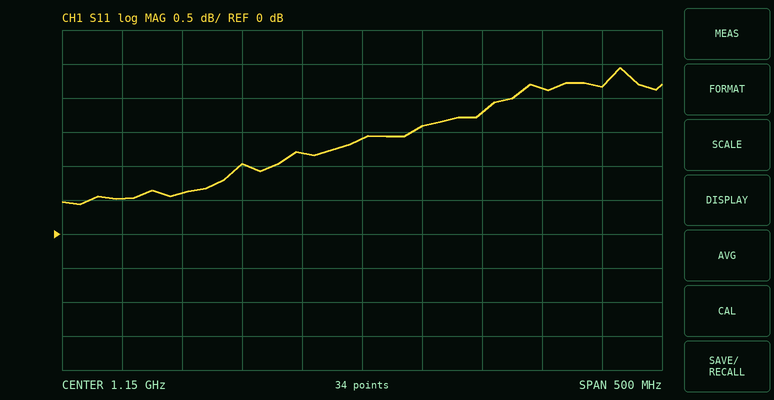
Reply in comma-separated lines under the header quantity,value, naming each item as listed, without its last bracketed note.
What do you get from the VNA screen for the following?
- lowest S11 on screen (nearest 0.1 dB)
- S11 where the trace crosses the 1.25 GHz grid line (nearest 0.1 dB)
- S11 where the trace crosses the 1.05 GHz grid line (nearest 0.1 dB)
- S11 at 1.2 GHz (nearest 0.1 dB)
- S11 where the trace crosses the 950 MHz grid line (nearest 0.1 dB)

quantity,value
lowest S11 on screen,0.4 dB
S11 where the trace crosses the 1.25 GHz grid line,1.8 dB
S11 where the trace crosses the 1.05 GHz grid line,1.0 dB
S11 at 1.2 GHz,1.6 dB
S11 where the trace crosses the 950 MHz grid line,0.5 dB
